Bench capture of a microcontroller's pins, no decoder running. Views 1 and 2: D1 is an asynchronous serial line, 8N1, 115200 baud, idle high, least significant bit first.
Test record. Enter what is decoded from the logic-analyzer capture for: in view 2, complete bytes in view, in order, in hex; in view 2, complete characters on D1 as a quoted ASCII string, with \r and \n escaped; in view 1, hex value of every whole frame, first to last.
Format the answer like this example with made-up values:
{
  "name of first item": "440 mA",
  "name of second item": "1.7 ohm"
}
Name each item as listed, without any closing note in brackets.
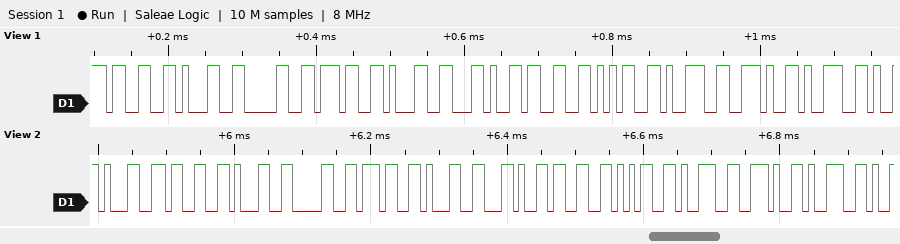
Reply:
{
  "in view 2, complete bytes in view, in order, in hex": "31 33 31 30 37 31 2C 33 35 39 2E 39",
  "in view 2, complete characters on D1 as a quoted ASCII string, with \\r and \\n escaped": "\"131071,359.9\"",
  "in view 1, hex value of every whole frame, first to last": "33 31 30 37 31 2C 33 35 39 2E 39"
}
